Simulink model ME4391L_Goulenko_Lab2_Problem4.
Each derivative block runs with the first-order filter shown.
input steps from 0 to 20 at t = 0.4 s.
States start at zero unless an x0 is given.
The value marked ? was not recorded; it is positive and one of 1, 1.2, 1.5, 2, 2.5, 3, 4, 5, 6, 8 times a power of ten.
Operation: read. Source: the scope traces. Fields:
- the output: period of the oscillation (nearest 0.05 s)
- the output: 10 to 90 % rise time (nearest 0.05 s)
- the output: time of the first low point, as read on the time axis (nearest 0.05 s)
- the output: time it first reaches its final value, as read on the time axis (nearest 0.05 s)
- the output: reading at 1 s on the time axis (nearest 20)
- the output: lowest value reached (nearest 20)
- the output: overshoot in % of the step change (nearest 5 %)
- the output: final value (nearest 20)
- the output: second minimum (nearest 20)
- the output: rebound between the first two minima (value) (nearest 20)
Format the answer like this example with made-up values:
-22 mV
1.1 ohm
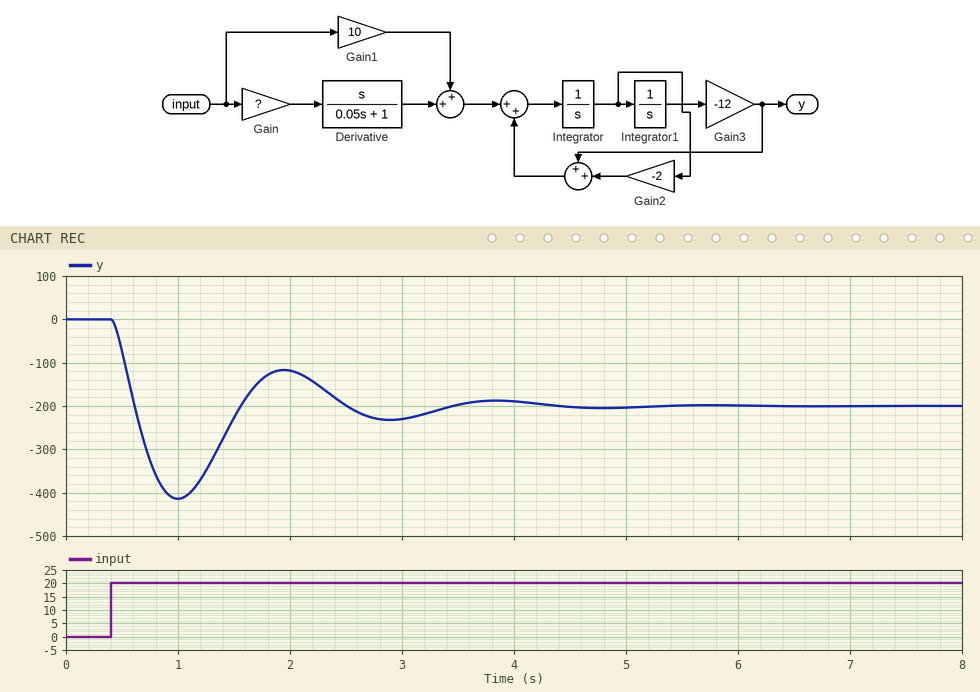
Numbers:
1.90 s
0.15 s
1.00 s
0.60 s
-420
-420
105 %
-200
-240
-120
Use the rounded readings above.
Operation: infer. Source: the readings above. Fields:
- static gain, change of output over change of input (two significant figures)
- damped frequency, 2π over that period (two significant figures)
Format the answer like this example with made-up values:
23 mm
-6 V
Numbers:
-10
3.3 rad/s
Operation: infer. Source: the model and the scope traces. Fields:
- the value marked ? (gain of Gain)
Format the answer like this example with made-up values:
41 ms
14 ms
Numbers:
5
